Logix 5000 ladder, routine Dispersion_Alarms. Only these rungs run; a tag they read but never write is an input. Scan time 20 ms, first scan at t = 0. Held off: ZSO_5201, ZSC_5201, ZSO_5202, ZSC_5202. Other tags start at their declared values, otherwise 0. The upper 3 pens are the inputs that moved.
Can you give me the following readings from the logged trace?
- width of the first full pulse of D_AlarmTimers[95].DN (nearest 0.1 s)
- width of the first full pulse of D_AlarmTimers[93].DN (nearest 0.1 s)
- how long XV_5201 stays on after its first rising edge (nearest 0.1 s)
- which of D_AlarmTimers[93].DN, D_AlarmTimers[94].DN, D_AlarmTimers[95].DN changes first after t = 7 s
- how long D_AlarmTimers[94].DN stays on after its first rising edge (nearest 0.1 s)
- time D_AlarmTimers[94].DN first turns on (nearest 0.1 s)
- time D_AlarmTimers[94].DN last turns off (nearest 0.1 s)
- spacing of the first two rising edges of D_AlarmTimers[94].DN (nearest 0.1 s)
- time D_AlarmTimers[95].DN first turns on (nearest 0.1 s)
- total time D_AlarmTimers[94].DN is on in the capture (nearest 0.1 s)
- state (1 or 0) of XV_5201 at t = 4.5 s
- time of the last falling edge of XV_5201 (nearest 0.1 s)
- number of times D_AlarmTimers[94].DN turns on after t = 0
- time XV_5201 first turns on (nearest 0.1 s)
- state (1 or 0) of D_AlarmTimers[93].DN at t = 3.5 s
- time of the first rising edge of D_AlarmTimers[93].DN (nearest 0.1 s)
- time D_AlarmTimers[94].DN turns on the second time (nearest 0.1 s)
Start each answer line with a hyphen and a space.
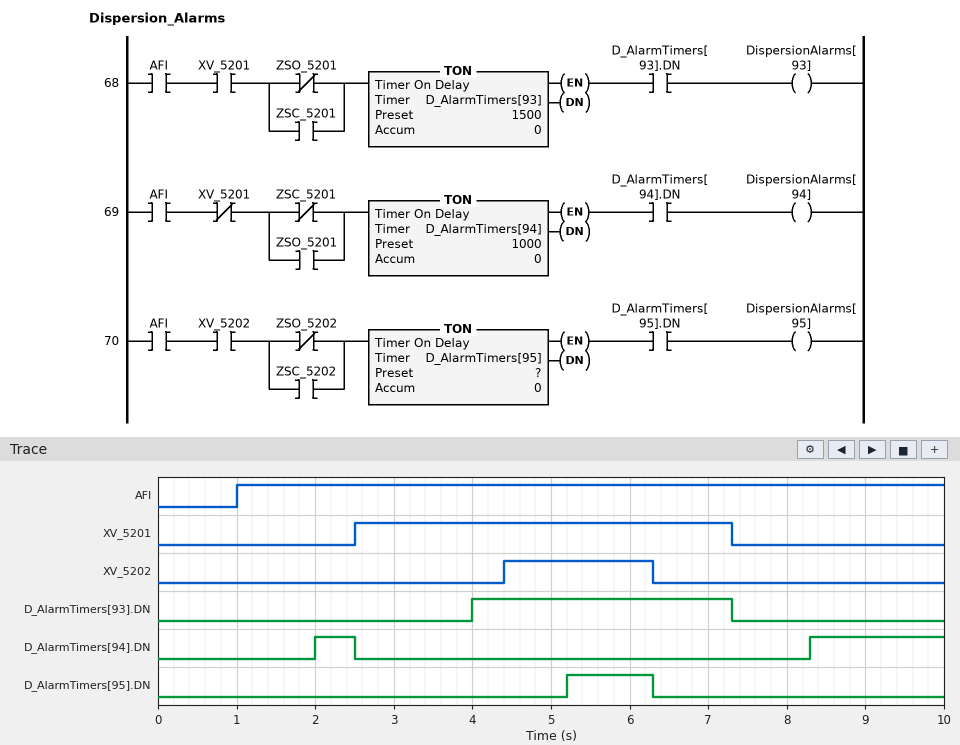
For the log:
- 1.1 s
- 3.3 s
- 4.8 s
- D_AlarmTimers[93].DN
- 0.5 s
- 2.0 s
- 2.5 s
- 6.3 s
- 5.2 s
- 2.2 s
- 1
- 7.3 s
- 2
- 2.5 s
- 0
- 4.0 s
- 8.3 s
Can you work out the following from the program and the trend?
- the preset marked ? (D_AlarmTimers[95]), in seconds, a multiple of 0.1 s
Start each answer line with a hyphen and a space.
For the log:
- 0.8 s
